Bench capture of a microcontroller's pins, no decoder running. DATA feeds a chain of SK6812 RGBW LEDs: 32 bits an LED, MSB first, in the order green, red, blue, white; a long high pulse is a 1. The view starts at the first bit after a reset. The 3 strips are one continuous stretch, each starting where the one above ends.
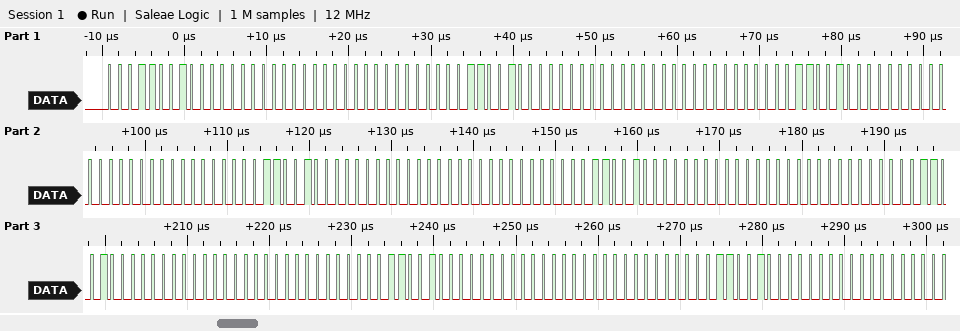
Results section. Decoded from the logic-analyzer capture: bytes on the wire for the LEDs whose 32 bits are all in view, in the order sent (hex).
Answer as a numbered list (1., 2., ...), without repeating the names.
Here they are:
1. 19 00 00 00 19 00 00 00 19 00 00 00 19 00 00 00 19 00 00 00 19 00 00 00 19 00 00 00
